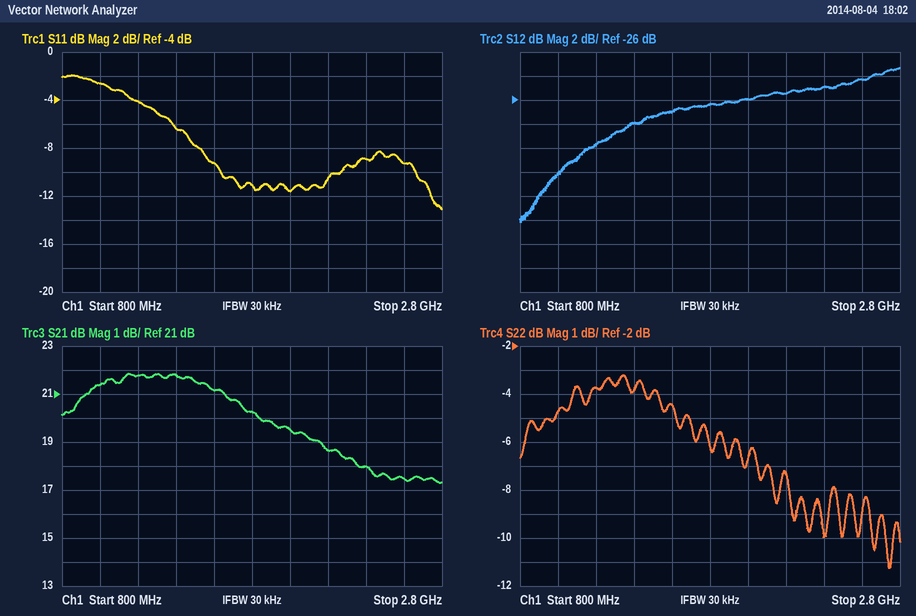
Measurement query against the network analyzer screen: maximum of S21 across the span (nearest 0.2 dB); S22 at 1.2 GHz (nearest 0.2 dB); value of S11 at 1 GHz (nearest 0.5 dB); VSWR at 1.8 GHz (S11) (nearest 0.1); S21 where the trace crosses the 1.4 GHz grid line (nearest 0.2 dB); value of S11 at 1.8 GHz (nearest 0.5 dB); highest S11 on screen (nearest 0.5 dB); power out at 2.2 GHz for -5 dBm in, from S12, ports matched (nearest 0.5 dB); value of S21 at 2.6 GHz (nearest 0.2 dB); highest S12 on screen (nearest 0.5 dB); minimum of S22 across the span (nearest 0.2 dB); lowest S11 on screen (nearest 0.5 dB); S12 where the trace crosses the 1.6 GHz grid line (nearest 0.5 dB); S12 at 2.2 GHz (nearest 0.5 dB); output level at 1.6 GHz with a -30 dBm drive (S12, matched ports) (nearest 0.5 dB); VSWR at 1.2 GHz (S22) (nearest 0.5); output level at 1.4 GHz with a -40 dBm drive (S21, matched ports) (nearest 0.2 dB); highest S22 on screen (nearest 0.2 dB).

21.8 dB
-3.8 dB
-2.5 dB
1.8
21.8 dB
-11.0 dB
-2.0 dB
-30.5 dBm
17.4 dB
-23.5 dB
-11.2 dB
-13.0 dB
-27.0 dB
-25.5 dB
-57.0 dBm
4.5
-18.2 dBm
-3.2 dB
